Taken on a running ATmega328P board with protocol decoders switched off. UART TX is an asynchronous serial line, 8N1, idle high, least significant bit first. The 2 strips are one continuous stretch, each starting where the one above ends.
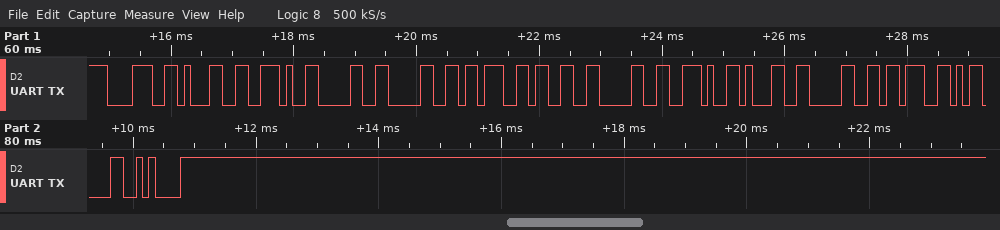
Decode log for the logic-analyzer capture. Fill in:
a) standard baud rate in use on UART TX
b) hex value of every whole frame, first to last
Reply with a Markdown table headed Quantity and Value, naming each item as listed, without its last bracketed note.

| Quantity | Value |
|---|---|
| standard baud rate in use on UART TX | 9600 baud |
| hex value of every whole frame, first to last | 0x38 0x31 0x2E 0x30 0x30 0x3B 0x33 0x30 0x2E 0x31 0x30 0x3B 0x0D 0x0A |
